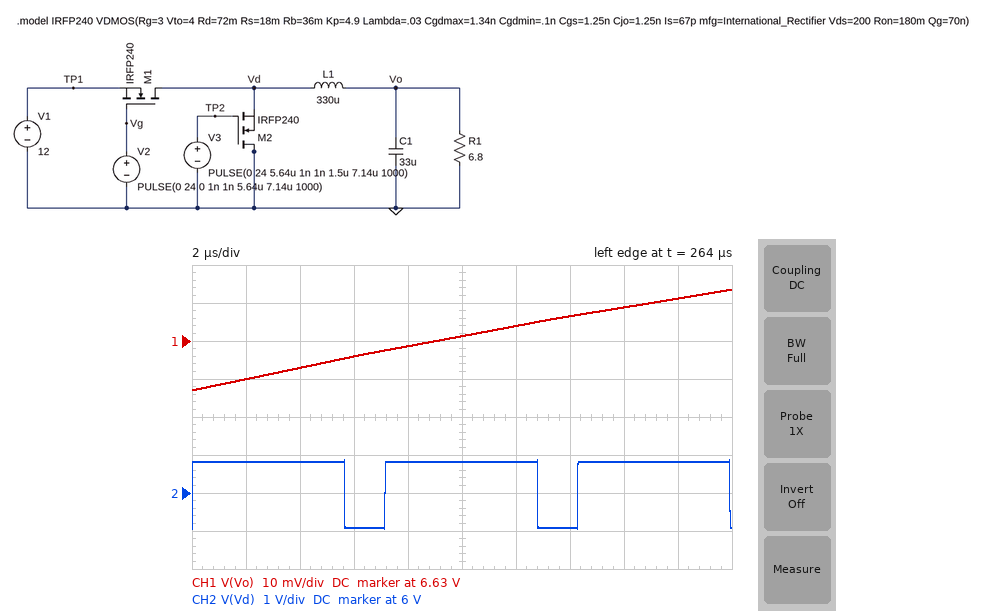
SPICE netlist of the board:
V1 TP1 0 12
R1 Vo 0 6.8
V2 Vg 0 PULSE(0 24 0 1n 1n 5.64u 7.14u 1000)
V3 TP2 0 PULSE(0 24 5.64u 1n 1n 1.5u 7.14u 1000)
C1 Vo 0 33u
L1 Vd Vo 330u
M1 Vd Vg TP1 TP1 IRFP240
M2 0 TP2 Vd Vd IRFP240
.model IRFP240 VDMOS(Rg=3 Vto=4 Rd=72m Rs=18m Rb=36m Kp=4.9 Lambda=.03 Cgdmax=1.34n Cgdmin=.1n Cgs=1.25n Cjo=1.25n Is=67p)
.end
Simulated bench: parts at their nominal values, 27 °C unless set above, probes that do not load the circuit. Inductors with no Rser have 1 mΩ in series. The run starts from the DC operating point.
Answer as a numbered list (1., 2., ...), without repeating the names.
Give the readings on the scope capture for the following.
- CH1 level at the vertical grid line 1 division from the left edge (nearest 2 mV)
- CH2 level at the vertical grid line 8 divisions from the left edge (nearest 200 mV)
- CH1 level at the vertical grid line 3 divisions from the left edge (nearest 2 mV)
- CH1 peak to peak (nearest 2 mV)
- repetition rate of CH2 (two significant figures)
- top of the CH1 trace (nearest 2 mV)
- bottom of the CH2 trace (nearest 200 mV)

1. 6.620 V
2. 6.8 V
3. 6.626 V
4. 26 mV
5. 140 kHz
6. 6.644 V
7. 5.0 V
